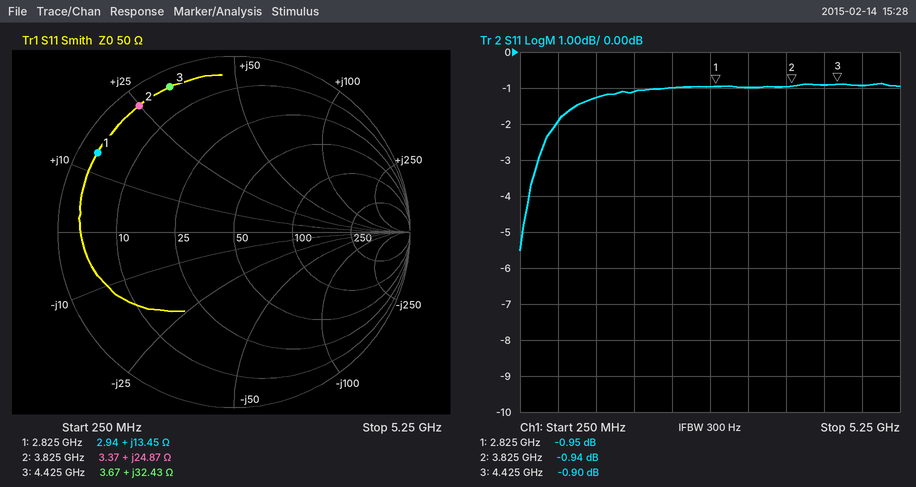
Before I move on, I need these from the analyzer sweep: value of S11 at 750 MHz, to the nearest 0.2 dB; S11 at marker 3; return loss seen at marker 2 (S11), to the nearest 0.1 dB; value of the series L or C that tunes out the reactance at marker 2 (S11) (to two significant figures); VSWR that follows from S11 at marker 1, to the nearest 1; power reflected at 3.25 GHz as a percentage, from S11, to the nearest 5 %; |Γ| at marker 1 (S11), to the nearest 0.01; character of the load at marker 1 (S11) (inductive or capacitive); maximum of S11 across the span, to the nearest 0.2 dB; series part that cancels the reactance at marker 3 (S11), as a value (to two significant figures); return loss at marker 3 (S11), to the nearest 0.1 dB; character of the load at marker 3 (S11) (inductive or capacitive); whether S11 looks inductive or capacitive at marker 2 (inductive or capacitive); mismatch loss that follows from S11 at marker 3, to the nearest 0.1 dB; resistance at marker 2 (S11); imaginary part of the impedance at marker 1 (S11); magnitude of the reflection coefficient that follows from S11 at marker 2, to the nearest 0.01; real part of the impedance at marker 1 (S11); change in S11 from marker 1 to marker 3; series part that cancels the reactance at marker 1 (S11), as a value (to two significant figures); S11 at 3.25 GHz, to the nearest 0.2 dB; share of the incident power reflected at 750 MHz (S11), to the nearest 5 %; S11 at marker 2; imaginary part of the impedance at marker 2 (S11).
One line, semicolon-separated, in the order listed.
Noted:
-2.0 dB; -0.90 dB; 0.9 dB; 1.7 pF; 18; 80 %; 0.90; inductive; -0.8 dB; 1.1 pF; 0.9 dB; inductive; inductive; 7.3 dB; 3.37 Ω; +13.45 Ω; 0.90; 2.94 Ω; 0.05 dB; 4.2 pF; -1.0 dB; 65 %; -0.94 dB; +24.87 Ω
